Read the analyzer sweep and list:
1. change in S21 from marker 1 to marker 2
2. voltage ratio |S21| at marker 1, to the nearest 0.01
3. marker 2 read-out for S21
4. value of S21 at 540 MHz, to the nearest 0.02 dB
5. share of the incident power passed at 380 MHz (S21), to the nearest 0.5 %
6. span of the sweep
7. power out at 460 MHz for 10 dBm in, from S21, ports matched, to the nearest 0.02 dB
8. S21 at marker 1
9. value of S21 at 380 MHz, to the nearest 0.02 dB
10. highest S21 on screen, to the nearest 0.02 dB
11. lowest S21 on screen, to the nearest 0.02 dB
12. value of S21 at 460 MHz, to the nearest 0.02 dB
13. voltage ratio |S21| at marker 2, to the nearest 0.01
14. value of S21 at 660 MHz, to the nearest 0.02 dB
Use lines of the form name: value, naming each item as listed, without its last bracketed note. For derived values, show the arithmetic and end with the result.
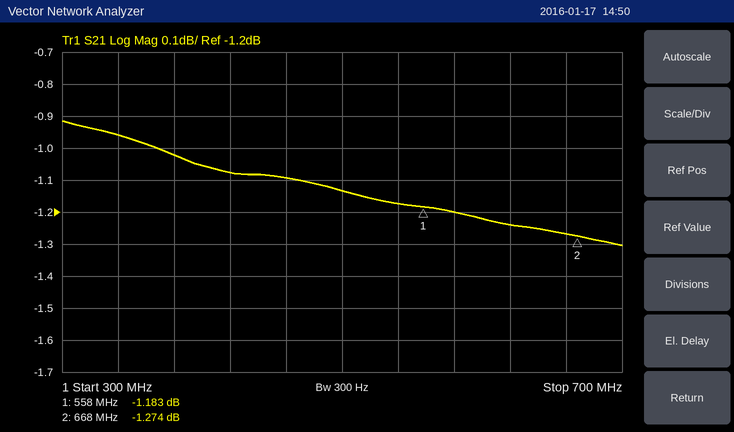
change in S21 from marker 1 to marker 2: -1.274 − (-1.183) = -0.091 dB
voltage ratio |S21| at marker 1, to the nearest 0.01: 10^(-1.183/20) ≈ 0.87
marker 2 read-out for S21: -1.274 dB
value of S21 at 540 MHz, to the nearest 0.02 dB: -1.18 dB
share of the incident power passed at 380 MHz (S21), to the nearest 0.5 %: 10^(-1.02/10) ≈ 79.1 %, so 79.0 % to the nearest 0.5 %
span of the sweep: 400 MHz
power out at 460 MHz for 10 dBm in, from S21, ports matched, to the nearest 0.02 dB: 10 dBm + (-1.10 dB) = 8.90 dBm
S21 at marker 1: -1.183 dB
value of S21 at 380 MHz, to the nearest 0.02 dB: -1.02 dB
highest S21 on screen, to the nearest 0.02 dB: -0.92 dB
lowest S21 on screen, to the nearest 0.02 dB: -1.30 dB
value of S21 at 460 MHz, to the nearest 0.02 dB: -1.10 dB
voltage ratio |S21| at marker 2, to the nearest 0.01: 10^(-1.274/20) ≈ 0.86
value of S21 at 660 MHz, to the nearest 0.02 dB: -1.26 dB
